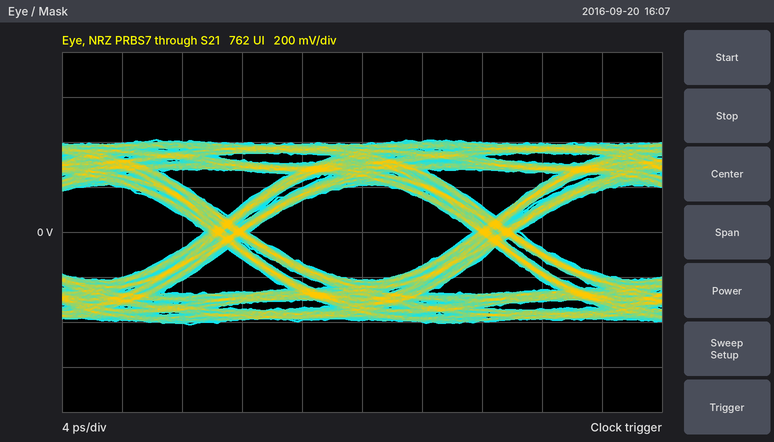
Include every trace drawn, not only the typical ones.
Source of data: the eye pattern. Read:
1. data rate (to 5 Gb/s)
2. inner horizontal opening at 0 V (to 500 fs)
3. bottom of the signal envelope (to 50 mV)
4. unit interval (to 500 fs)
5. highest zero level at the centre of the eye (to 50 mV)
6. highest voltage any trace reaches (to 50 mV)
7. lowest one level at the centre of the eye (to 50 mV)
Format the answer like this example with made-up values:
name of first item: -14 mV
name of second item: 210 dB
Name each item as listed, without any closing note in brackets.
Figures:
data rate: 55 Gb/s
inner horizontal opening at 0 V: 15.0 ps
bottom of the signal envelope: -400 mV
unit interval: 18.0 ps
highest zero level at the centre of the eye: -200 mV
highest voltage any trace reaches: 400 mV
lowest one level at the centre of the eye: 200 mV
